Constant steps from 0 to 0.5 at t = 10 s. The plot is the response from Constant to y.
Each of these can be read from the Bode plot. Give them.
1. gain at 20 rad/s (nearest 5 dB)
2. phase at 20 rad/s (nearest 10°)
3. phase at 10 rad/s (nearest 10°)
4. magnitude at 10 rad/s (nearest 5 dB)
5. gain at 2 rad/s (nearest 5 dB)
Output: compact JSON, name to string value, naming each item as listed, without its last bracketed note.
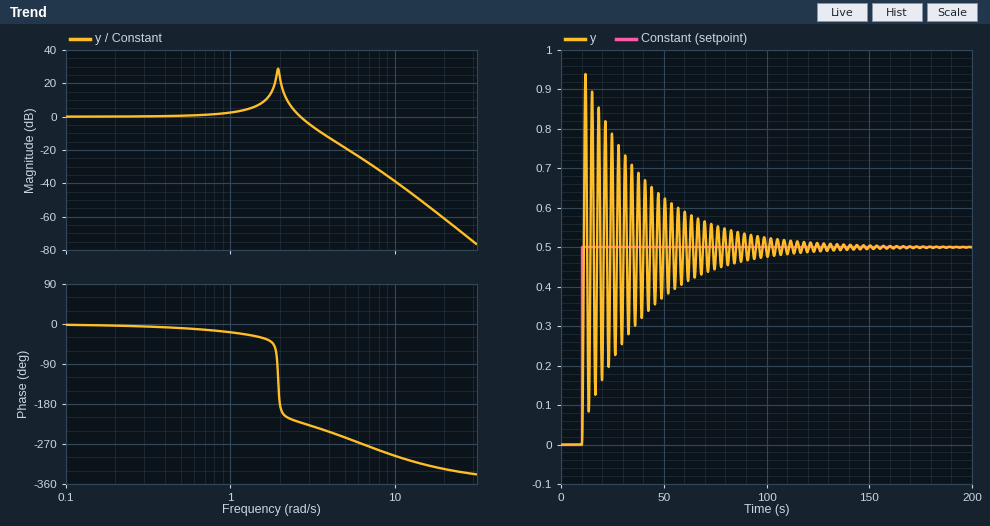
{"gain at 20 rad/s": "-60 dB", "phase at 20 rad/s": "-330°", "phase at 10 rad/s": "-300°", "magnitude at 10 rad/s": "-40 dB", "gain at 2 rad/s": "25 dB"}
